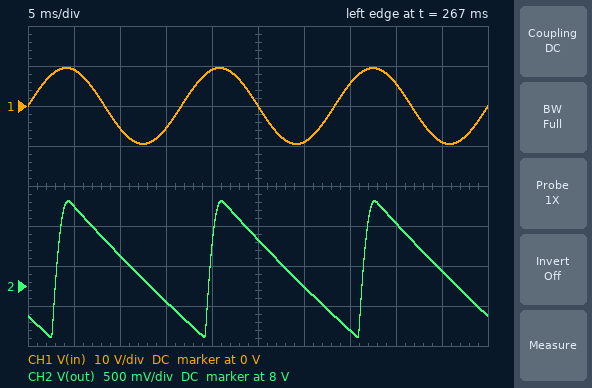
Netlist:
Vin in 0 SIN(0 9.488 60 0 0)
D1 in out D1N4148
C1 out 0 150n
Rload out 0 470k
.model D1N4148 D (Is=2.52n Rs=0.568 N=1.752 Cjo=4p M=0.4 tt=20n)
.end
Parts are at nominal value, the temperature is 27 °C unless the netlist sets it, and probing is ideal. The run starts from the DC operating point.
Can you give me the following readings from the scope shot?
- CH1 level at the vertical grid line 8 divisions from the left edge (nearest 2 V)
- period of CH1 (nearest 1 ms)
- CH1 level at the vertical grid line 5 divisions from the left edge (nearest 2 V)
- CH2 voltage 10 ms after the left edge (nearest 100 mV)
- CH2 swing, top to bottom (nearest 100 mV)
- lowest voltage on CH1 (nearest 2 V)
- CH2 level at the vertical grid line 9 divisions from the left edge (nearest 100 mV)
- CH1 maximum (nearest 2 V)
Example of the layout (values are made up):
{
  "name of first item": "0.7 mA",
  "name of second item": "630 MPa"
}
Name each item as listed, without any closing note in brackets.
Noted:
{
  "CH1 level at the vertical grid line 8 divisions from the left edge": "6 V",
  "period of CH1": "17 ms",
  "CH1 level at the vertical grid line 5 divisions from the left edge": "0 V",
  "CH2 voltage 10 ms after the left edge": "8.4 V",
  "CH2 swing, top to bottom": "1.7 V",
  "lowest voltage on CH1": "-10 V",
  "CH2 level at the vertical grid line 9 divisions from the left edge": "8.2 V",
  "CH1 maximum": "10 V"
}
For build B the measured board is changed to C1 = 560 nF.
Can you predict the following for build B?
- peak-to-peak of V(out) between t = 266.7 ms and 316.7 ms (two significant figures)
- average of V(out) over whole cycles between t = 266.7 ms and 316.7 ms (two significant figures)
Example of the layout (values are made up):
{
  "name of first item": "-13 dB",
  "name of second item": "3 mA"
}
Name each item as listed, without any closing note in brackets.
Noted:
{
  "peak-to-peak of V(out) between t = 266.7 ms and 316.7 ms": "510 mV",
  "average of V(out) over whole cycles between t = 266.7 ms and 316.7 ms": "8.8 V"
}
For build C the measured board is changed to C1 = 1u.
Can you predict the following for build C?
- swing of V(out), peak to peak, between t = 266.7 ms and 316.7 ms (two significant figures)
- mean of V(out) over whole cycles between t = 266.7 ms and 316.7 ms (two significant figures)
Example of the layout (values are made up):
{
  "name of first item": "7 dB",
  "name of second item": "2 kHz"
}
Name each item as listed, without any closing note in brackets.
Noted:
{
  "swing of V(out), peak to peak, between t = 266.7 ms and 316.7 ms": "290 mV",
  "mean of V(out) over whole cycles between t = 266.7 ms and 316.7 ms": "8.9 V"
}
